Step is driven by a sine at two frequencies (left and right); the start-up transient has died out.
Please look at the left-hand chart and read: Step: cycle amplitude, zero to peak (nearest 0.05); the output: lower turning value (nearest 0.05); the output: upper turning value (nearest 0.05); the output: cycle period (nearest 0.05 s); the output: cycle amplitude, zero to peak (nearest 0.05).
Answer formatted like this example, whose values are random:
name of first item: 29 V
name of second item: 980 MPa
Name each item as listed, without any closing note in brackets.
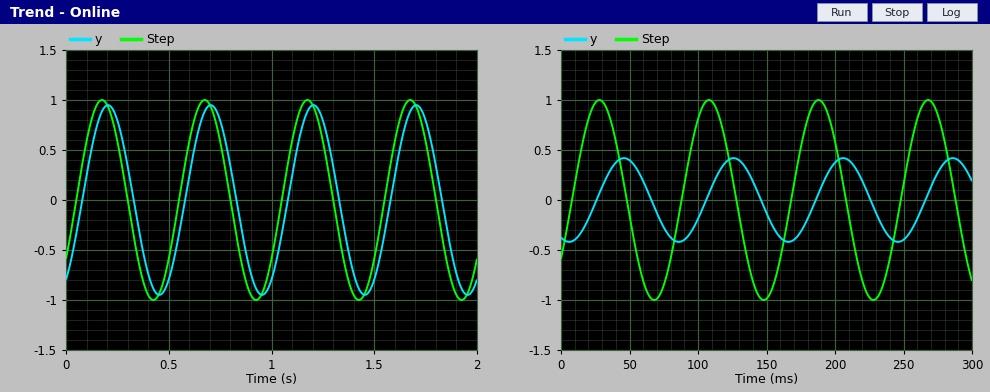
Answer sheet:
Step: cycle amplitude, zero to peak: 1.00
the output: lower turning value: -0.95
the output: upper turning value: 0.95
the output: cycle period: 0.50 s
the output: cycle amplitude, zero to peak: 0.95
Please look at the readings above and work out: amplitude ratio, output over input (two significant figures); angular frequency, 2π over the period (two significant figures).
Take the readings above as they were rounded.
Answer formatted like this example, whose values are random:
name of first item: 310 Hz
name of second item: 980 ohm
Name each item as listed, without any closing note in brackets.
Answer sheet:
amplitude ratio, output over input: 0.95
angular frequency, 2π over the period: 13 rad/s
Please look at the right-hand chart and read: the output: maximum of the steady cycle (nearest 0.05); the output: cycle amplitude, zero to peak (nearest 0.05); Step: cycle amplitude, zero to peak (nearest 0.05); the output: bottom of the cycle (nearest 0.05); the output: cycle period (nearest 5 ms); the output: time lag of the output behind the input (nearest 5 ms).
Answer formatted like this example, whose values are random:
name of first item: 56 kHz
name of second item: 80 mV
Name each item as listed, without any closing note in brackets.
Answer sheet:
the output: maximum of the steady cycle: 0.40
the output: cycle amplitude, zero to peak: 0.40
Step: cycle amplitude, zero to peak: 1.00
the output: bottom of the cycle: -0.40
the output: cycle period: 80 ms
the output: time lag of the output behind the input: 20 ms
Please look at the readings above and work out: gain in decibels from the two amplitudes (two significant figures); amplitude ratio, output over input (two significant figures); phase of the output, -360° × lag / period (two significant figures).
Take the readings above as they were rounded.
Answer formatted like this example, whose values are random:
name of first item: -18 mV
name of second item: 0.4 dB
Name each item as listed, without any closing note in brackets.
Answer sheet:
gain in decibels from the two amplitudes: -8.0 dB
amplitude ratio, output over input: 0.40
phase of the output, -360° × lag / period: -90°
